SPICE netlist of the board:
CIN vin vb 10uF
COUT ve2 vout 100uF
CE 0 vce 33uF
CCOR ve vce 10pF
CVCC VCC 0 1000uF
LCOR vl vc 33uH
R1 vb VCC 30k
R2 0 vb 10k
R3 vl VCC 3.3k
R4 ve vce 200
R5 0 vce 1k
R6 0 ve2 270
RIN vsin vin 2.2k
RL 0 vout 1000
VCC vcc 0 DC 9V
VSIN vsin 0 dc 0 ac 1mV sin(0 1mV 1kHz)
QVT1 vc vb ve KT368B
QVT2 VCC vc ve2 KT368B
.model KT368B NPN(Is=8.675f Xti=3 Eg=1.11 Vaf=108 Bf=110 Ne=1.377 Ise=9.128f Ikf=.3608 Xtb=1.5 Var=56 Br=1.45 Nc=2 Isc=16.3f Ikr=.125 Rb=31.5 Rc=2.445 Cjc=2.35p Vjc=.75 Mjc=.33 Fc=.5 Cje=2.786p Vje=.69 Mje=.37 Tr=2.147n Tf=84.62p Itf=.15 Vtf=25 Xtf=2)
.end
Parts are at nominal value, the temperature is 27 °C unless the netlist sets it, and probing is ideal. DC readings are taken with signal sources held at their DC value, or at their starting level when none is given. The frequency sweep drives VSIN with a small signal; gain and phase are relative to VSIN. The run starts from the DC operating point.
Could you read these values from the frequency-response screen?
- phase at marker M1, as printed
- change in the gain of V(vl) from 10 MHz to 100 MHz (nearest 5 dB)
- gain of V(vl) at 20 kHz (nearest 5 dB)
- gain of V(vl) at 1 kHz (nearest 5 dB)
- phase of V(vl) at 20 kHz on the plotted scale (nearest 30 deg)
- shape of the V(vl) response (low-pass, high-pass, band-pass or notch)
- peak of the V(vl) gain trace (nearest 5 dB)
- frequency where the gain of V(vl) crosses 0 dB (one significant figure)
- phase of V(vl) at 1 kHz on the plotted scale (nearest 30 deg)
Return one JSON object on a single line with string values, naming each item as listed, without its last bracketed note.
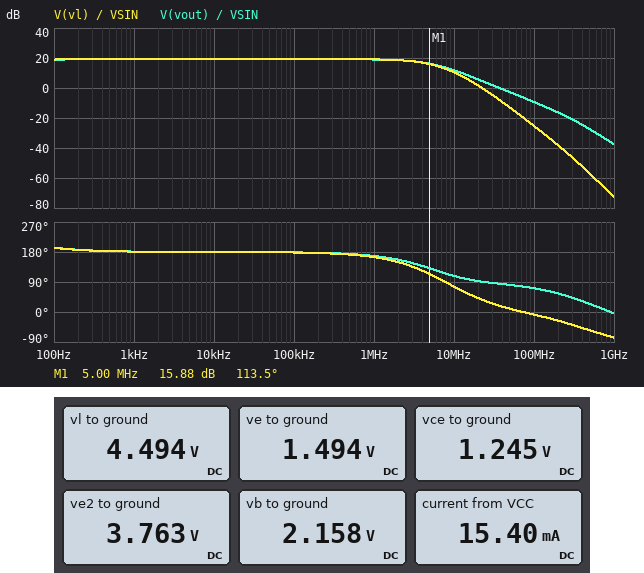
{"phase at marker M1, as printed": "113.5 deg", "change in the gain of V(vl) from 10 MHz to 100 MHz": "-35 dB", "gain of V(vl) at 20 kHz": "20 dB", "gain of V(vl) at 1 kHz": "20 dB", "phase of V(vl) at 20 kHz on the plotted scale": "180 deg", "shape of the V(vl) response": "low-pass", "peak of the V(vl) gain trace": "20 dB", "frequency where the gain of V(vl) crosses 0 dB": "20 MHz", "phase of V(vl) at 1 kHz on the plotted scale": "180 deg"}
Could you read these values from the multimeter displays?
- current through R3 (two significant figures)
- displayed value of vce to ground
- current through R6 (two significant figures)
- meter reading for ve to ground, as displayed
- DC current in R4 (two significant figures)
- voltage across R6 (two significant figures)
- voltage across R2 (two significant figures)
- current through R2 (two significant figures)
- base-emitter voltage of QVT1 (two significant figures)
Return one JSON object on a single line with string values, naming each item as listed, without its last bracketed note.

{"current through R3": "1.4 mA", "displayed value of vce to ground": "1.245 V", "current through R6": "14 mA", "meter reading for ve to ground, as displayed": "1.494 V", "DC current in R4": "1.2 mA", "voltage across R6": "3.8 V", "voltage across R2": "2.2 V", "current through R2": "220 µA", "base-emitter voltage of QVT1": "660 mV"}
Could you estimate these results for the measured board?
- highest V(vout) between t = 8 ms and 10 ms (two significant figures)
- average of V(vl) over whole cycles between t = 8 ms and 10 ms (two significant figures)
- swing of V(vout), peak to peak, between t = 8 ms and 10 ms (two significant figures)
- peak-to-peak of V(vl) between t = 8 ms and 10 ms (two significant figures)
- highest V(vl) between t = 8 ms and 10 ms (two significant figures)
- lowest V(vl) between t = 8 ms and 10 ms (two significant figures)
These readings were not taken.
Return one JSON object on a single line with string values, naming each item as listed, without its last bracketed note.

{"highest V(vout) between t = 8 ms and 10 ms": "9.1 mV", "average of V(vl) over whole cycles between t = 8 ms and 10 ms": "4.5 V", "swing of V(vout), peak to peak, between t = 8 ms and 10 ms": "18 mV", "peak-to-peak of V(vl) between t = 8 ms and 10 ms": "18 mV", "highest V(vl) between t = 8 ms and 10 ms": "4.5 V", "lowest V(vl) between t = 8 ms and 10 ms": "4.5 V"}
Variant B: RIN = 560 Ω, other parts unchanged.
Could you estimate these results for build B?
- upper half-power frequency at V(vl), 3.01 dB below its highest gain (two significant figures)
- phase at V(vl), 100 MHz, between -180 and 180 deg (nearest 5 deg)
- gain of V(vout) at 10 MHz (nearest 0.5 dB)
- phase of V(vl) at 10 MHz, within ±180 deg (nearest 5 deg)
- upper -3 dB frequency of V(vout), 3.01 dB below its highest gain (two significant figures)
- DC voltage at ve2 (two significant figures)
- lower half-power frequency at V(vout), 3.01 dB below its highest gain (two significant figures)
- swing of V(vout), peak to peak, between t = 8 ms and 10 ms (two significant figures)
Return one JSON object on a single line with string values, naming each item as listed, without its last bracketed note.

{"upper half-power frequency at V(vl), 3.01 dB below its highest gain": "11 MHz", "phase at V(vl), 100 MHz, between -180 and 180 deg": "5 deg", "gain of V(vout) at 10 MHz": "20.5 dB", "phase of V(vl) at 10 MHz, within ±180 deg": "100 deg", "upper -3 dB frequency of V(vout), 3.01 dB below its highest gain": "14 MHz", "DC voltage at ve2": "3.8 V", "lower half-power frequency at V(vout), 3.01 dB below its highest gain": "27 Hz", "swing of V(vout), peak to peak, between t = 8 ms and 10 ms": "23 mV"}
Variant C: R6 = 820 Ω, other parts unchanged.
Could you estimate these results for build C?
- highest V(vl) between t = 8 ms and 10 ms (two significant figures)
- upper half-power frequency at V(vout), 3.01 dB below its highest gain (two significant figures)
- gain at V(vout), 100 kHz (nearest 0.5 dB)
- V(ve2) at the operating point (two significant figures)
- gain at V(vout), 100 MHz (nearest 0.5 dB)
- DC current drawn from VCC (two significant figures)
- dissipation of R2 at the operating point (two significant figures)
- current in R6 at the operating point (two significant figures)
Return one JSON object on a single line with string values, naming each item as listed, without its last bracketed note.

{"highest V(vl) between t = 8 ms and 10 ms": "4.8 V", "upper half-power frequency at V(vout), 3.01 dB below its highest gain": "5.0 MHz", "gain at V(vout), 100 kHz": "20.0 dB", "V(ve2) at the operating point": "4.1 V", "gain at V(vout), 100 MHz": "-9.0 dB", "DC current drawn from VCC": "6.4 mA", "dissipation of R2 at the operating point": "470 µW", "current in R6 at the operating point": "5.0 mA"}
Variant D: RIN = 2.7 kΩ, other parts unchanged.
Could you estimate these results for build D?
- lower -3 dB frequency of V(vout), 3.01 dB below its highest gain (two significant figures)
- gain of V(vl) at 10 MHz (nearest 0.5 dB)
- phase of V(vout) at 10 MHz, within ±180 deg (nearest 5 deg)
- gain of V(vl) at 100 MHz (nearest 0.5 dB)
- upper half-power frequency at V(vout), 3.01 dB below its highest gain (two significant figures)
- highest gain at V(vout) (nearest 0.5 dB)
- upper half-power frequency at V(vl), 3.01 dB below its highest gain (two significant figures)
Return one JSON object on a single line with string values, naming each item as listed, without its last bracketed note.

{"lower -3 dB frequency of V(vout), 3.01 dB below its highest gain": "24 Hz", "gain of V(vl) at 10 MHz": "9.0 dB", "phase of V(vout) at 10 MHz, within ±180 deg": "105 deg", "gain of V(vl) at 100 MHz": "-27.0 dB", "upper half-power frequency at V(vout), 3.01 dB below its highest gain": "4.3 MHz", "highest gain at V(vout)": "18.5 dB", "upper half-power frequency at V(vl), 3.01 dB below its highest gain": "4.1 MHz"}
